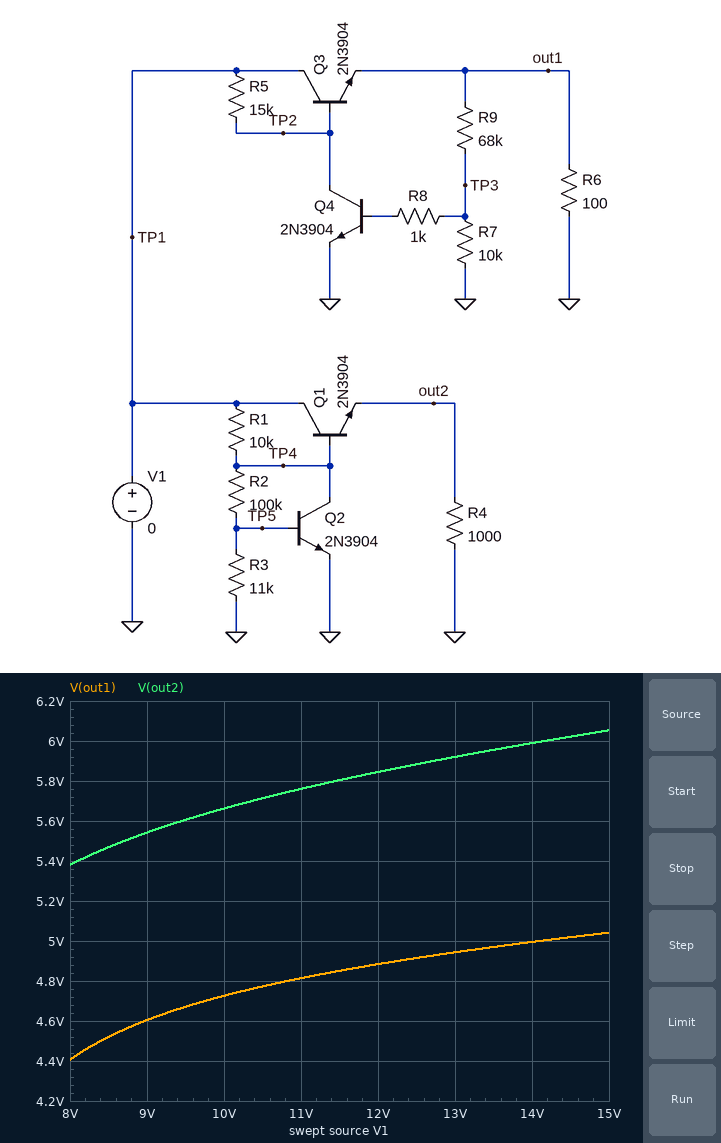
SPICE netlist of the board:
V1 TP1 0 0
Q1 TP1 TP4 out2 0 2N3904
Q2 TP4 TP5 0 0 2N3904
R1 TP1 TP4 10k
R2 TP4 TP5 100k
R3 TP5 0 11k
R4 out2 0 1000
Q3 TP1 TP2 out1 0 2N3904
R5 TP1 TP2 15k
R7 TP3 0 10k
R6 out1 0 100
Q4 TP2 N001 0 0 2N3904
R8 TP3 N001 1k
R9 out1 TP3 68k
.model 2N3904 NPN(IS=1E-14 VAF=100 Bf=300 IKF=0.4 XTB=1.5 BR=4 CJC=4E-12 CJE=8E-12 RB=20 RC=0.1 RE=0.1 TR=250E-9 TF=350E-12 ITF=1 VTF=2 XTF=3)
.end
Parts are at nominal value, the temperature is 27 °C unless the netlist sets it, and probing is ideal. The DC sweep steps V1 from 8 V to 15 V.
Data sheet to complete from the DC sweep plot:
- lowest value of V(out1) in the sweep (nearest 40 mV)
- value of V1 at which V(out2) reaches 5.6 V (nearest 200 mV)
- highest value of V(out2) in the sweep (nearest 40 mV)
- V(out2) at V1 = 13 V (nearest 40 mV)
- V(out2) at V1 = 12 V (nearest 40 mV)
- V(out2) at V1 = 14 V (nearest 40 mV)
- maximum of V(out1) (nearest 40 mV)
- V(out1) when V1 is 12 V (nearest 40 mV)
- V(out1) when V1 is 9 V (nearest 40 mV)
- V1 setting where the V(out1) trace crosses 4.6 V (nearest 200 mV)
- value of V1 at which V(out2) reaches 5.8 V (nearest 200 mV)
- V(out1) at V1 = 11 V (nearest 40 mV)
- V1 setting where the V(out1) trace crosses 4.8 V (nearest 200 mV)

4.40 V
9.4 V
6.04 V
5.92 V
5.84 V
6.00 V
5.04 V
4.88 V
4.60 V
9.0 V
11.4 V
4.80 V
10.8 V
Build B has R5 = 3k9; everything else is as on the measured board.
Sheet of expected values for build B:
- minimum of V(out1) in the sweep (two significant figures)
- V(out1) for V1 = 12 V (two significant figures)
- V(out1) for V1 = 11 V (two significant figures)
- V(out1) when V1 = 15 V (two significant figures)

5.0 V
5.5 V
5.4 V
5.7 V
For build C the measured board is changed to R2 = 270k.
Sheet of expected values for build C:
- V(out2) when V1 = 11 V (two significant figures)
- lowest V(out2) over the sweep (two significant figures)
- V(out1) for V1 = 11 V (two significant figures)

9.6 V
6.8 V
4.8 V
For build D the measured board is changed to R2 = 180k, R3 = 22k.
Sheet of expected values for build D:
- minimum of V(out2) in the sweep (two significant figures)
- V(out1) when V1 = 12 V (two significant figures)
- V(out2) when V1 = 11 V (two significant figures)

5.0 V
4.9 V
5.4 V
